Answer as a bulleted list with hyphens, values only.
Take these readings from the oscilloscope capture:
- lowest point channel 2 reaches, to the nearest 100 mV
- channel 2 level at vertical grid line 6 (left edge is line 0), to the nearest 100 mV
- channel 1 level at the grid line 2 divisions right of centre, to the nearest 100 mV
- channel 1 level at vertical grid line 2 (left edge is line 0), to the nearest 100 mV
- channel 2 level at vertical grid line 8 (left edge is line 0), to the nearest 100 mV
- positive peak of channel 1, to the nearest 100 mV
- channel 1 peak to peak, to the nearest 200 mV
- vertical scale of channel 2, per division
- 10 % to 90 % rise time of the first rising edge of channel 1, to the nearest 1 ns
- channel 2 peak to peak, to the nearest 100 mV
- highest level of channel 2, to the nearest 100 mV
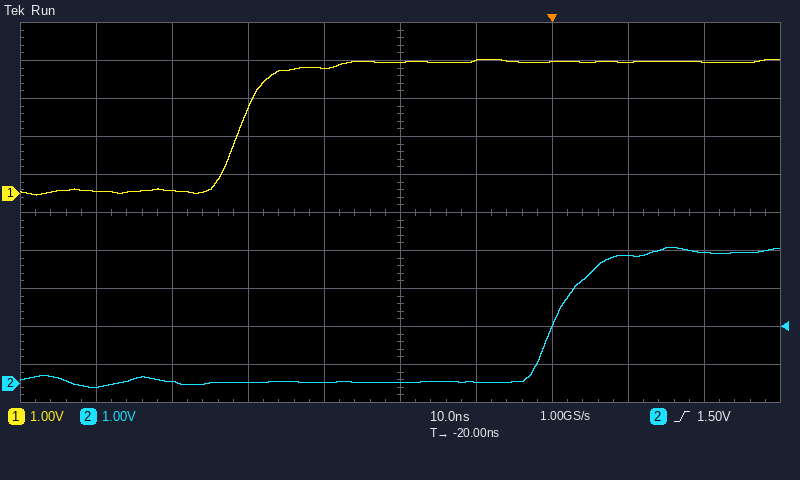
- -100 mV
- 0.0 V
- 3.5 V
- 100 mV
- 3.4 V
- 3.5 V
- 3.6 V
- 1 V
- 7 ns
- 3.7 V
- 3.6 V
